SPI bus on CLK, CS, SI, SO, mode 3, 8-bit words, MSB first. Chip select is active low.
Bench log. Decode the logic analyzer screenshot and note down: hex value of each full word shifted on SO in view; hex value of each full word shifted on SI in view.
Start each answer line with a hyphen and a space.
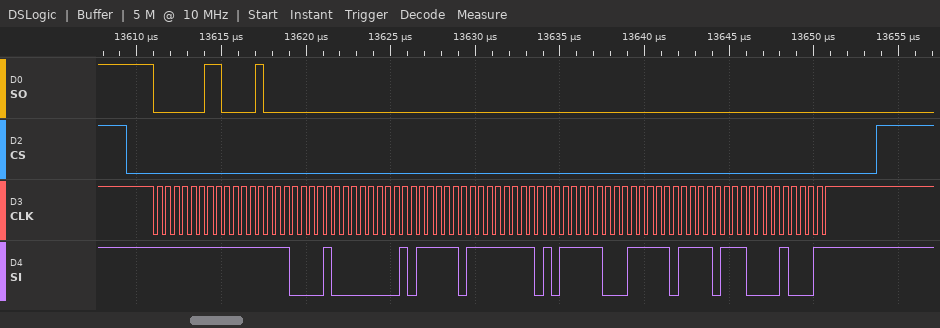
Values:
- 03, 08, 00, 00, 00, 00, 00, 00, 00, 00
- FF, FF, 08, 05, F7, FA, F8, FB, DC, 23
